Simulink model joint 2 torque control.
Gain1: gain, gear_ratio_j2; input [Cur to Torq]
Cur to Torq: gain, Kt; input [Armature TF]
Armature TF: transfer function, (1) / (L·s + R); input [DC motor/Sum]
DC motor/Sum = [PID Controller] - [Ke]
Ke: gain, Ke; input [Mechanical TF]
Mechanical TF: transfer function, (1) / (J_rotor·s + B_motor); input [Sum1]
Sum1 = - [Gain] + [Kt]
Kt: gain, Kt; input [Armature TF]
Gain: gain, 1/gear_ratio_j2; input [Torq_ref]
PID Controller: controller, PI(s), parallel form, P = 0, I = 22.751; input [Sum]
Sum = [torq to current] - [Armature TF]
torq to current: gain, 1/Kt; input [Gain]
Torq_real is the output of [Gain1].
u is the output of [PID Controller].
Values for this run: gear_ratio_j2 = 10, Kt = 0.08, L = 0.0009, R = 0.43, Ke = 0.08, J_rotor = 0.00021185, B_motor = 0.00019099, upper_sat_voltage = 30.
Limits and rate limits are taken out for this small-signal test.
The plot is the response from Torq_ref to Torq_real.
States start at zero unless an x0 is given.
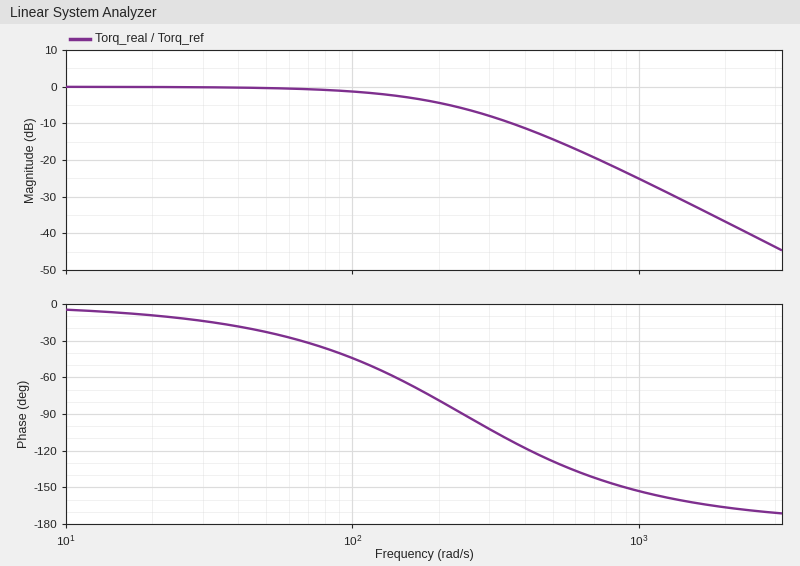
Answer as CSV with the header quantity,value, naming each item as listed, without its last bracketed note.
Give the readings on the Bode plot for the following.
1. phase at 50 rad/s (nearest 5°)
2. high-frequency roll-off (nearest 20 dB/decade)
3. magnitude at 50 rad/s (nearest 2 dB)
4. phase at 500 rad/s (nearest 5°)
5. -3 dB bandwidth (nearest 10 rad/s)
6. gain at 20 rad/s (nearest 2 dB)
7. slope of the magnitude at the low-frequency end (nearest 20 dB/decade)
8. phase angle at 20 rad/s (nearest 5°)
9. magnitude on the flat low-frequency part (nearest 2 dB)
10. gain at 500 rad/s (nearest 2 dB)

quantity,value
phase at 50 rad/s,-25°
high-frequency roll-off,-40 dB/decade
magnitude at 50 rad/s,0 dB
phase at 500 rad/s,-130°
-3 dB bandwidth,160 rad/s
gain at 20 rad/s,0 dB
slope of the magnitude at the low-frequency end,0 dB/decade
phase angle at 20 rad/s,-10°
magnitude on the flat low-frequency part,0 dB
gain at 500 rad/s,-14 dB
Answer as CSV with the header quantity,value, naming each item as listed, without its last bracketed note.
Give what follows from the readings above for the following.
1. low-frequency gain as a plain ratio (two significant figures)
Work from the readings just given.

quantity,value
low-frequency gain as a plain ratio,1.0
